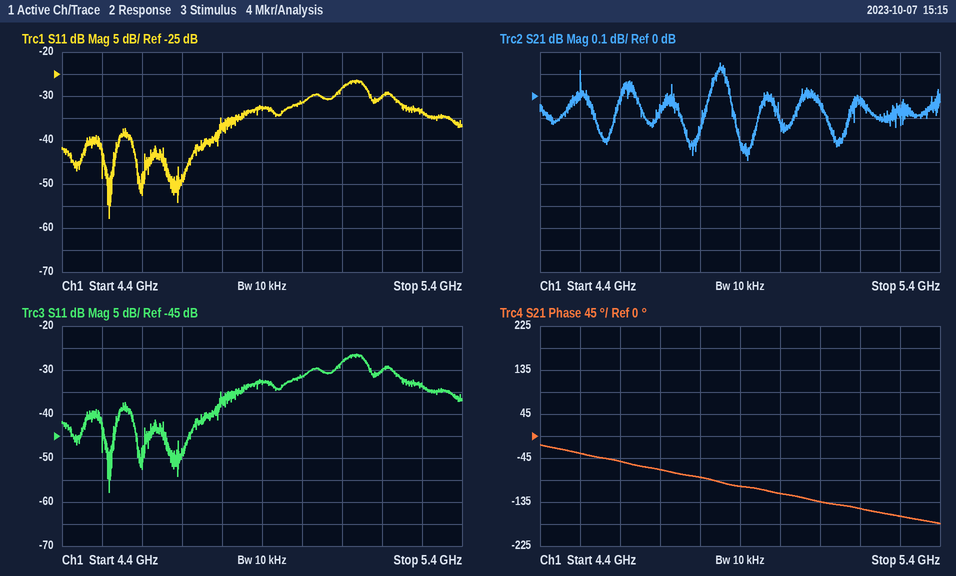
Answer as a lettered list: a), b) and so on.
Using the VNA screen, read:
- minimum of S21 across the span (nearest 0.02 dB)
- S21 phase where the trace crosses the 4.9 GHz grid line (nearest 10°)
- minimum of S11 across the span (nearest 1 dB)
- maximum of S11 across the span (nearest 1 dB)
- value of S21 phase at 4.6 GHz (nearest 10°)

a) -0.30 dB
b) -100°
c) -58 dB
d) -26 dB
e) -50°
